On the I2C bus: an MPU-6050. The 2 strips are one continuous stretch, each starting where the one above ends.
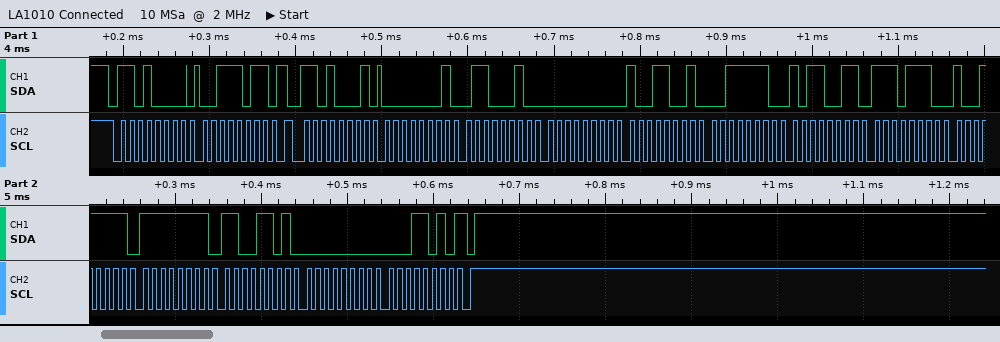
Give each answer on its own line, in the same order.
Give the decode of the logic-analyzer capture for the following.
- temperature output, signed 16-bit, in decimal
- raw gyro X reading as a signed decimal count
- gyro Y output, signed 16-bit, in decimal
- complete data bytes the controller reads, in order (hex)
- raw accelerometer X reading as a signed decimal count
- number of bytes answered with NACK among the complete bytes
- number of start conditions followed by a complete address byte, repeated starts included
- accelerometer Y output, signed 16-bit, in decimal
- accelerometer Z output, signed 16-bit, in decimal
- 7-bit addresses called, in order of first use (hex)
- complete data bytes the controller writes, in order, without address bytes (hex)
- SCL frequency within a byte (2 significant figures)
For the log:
-4449
-51
26
01 62 00 99 3E B3 EE 9F FF CD 00 1A
354
1
2
153
16051
0x68
3B
100 kHz
